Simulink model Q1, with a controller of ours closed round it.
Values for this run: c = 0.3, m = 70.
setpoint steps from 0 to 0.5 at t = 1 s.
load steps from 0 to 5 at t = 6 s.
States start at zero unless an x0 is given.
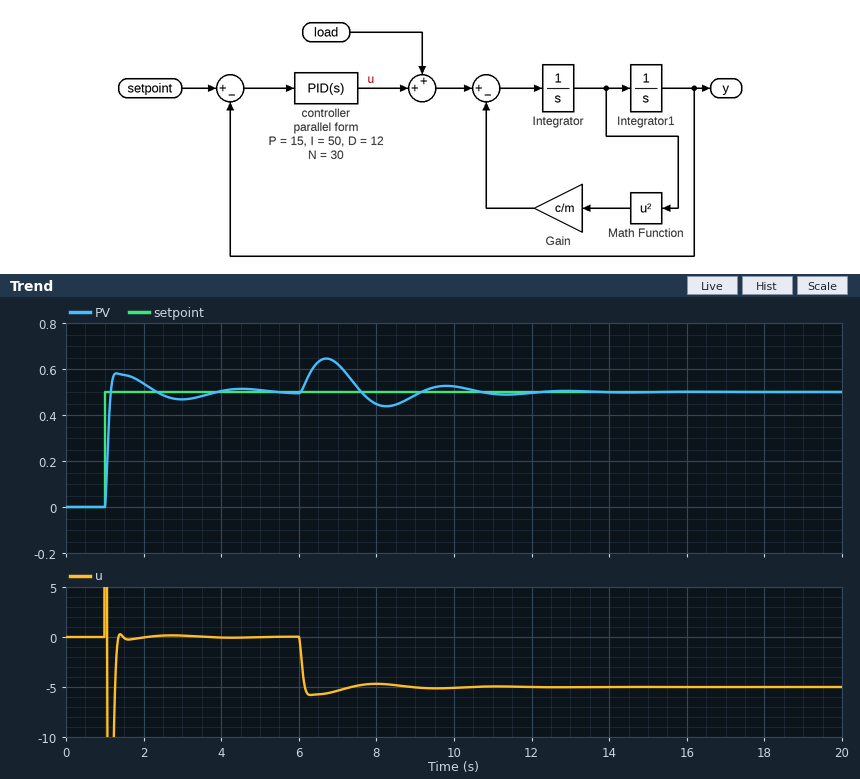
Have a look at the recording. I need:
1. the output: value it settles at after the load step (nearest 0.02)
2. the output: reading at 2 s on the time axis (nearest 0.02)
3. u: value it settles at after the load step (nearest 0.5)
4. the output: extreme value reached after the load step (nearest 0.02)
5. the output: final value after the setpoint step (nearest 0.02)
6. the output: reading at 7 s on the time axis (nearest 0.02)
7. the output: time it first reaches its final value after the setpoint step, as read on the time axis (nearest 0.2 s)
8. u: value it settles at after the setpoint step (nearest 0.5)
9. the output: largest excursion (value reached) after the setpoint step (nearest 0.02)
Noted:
0.50
0.54
-5.0
0.64
0.50
0.62
1.2 s
0.0
0.58
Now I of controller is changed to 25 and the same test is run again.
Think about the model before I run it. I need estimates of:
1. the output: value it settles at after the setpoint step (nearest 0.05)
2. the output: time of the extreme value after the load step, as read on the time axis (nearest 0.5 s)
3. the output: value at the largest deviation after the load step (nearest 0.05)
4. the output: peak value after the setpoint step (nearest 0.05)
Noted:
0.50
7.0 s
0.70
0.55
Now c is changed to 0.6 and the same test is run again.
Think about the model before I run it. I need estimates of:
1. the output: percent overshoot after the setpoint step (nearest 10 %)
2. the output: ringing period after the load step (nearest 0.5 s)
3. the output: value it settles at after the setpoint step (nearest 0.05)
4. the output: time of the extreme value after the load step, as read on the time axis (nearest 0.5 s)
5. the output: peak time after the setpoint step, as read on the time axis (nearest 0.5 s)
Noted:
20 %
3.0 s
0.50
6.5 s
1.5 s
